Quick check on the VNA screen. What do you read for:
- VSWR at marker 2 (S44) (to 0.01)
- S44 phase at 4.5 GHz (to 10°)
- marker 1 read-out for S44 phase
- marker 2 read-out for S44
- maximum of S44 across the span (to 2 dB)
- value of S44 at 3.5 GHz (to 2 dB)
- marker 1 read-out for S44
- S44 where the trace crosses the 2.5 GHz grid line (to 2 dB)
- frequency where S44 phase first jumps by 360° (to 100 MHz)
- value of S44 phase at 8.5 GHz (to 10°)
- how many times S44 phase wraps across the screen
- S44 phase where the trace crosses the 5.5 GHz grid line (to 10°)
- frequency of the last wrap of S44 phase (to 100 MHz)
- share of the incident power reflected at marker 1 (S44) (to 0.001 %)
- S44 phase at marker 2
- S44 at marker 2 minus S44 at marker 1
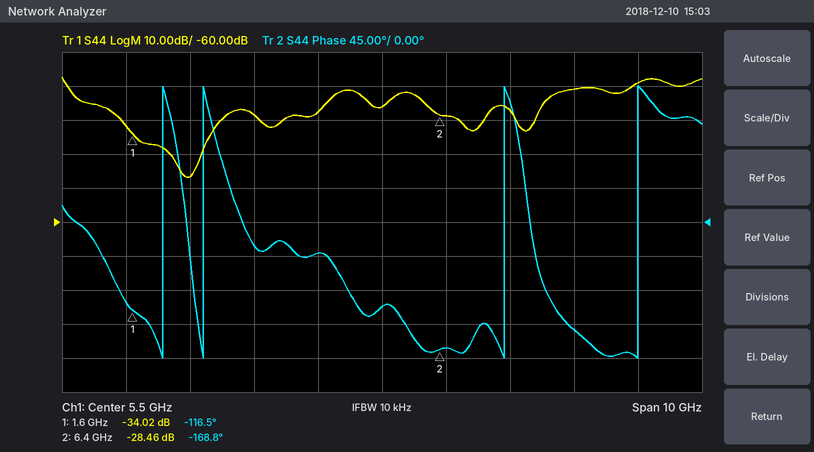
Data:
1.08
-40°
-116.5°
-28.46 dB
-18 dB
-28 dB
-34.02 dB
-46 dB
2.1 GHz
-140°
4
-110°
9.5 GHz
0.040 %
-168.8°
5.56 dB
